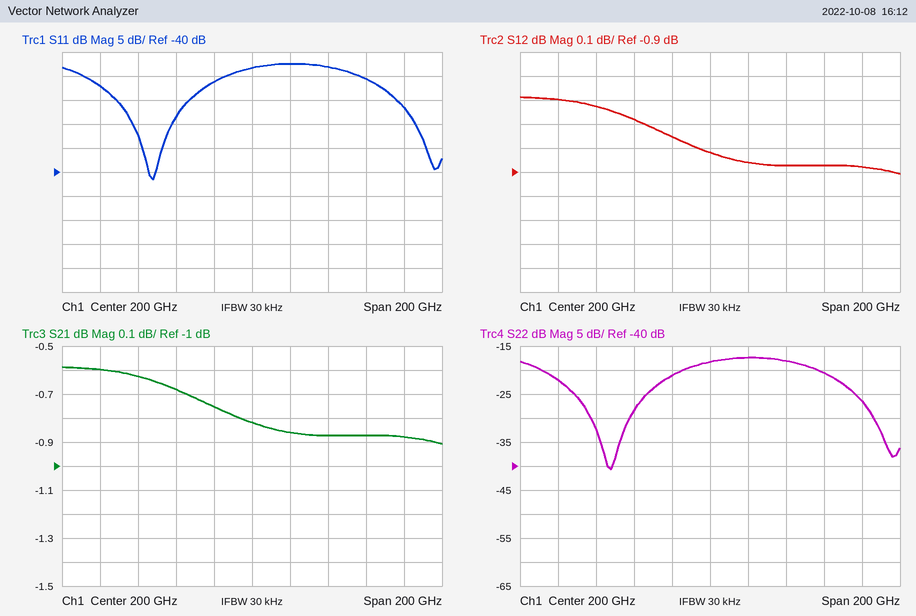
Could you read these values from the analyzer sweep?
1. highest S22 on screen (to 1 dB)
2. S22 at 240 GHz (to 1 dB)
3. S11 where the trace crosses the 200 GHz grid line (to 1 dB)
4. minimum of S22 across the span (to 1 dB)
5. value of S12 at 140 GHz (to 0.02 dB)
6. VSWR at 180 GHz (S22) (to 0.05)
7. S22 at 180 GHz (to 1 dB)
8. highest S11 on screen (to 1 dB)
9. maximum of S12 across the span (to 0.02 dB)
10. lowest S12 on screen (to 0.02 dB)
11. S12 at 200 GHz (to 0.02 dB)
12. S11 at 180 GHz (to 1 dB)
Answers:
-17 dB
-18 dB
-18 dB
-41 dB
-0.62 dB
1.20
-21 dB
-17 dB
-0.58 dB
-0.90 dB
-0.82 dB
-21 dB
